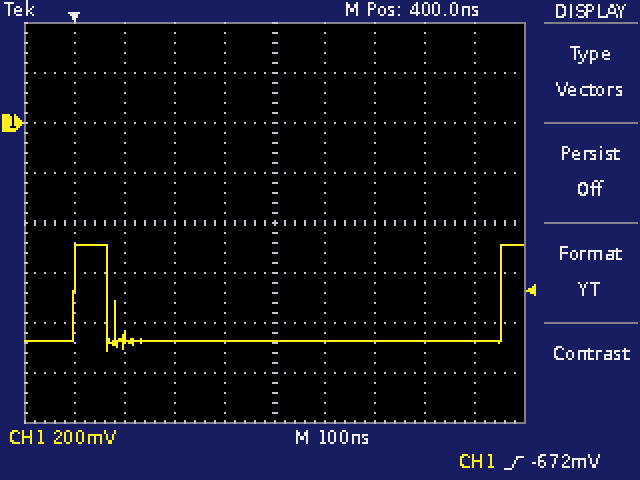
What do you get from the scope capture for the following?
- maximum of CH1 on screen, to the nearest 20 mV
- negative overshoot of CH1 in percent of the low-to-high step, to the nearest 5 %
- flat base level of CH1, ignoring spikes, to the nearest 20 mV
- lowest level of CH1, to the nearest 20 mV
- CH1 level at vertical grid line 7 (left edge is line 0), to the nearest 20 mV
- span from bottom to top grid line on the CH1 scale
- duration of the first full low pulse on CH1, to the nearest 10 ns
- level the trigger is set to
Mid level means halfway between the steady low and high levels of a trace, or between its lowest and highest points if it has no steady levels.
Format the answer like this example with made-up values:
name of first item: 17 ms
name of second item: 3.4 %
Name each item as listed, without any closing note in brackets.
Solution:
maximum of CH1 on screen, to the nearest 20 mV: -480 mV
negative overshoot of CH1 in percent of the low-to-high step, to the nearest 5 %: 10 %
flat base level of CH1, ignoring spikes, to the nearest 20 mV: -880 mV
lowest level of CH1, to the nearest 20 mV: -920 mV
CH1 level at vertical grid line 7 (left edge is line 0), to the nearest 20 mV: -880 mV
span from bottom to top grid line on the CH1 scale: 1.6 V
duration of the first full low pulse on CH1, to the nearest 10 ns: 790 ns
level the trigger is set to: -672 mV
